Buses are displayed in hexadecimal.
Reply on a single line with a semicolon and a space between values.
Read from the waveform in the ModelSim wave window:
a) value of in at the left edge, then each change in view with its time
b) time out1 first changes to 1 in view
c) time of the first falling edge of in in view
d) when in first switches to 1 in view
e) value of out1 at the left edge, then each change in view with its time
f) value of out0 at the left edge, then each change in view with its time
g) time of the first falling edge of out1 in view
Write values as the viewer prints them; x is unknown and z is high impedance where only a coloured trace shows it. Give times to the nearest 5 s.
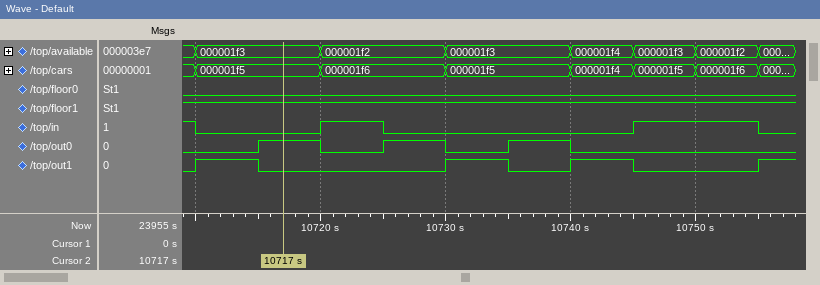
1, 0 at 10710 s, 1 at 10720 s, 0 at 10725 s, 1 at 10745 s, 0 at 10755 s; 10710 s; 10710 s; 10720 s; 0, 1 at 10710 s, 0 at 10715 s, 1 at 10730 s, 0 at 10735 s, 1 at 10740 s, 0 at 10745 s, 1 at 10755 s; 0, 1 at 10715 s, 0 at 10720 s, 1 at 10725 s, 0 at 10730 s, 1 at 10735 s, 0 at 10740 s; 10715 s
